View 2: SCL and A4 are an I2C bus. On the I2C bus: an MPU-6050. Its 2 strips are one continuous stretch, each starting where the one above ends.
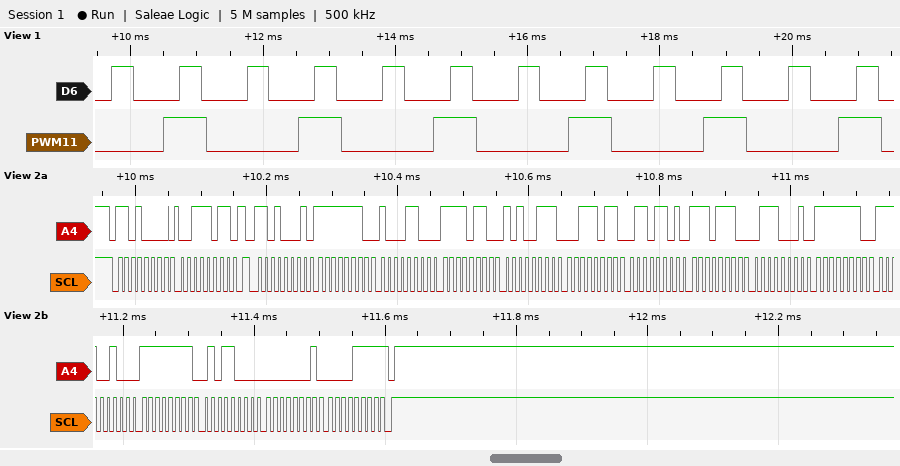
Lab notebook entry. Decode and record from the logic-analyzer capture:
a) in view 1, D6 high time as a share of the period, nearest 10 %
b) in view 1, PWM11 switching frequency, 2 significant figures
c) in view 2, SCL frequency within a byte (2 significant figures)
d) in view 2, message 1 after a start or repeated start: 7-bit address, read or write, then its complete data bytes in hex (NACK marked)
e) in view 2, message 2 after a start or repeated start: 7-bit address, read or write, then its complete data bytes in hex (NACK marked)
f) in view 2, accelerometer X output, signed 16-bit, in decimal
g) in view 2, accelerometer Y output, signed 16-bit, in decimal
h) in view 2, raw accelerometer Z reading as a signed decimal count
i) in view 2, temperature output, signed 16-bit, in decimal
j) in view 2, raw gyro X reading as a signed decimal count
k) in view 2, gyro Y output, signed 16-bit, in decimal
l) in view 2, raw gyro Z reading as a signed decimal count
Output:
30 %
490 Hz
100 kHz
0x68 write: 3B
0x68 read: FE 8C F6 A7 3B 6D EE 71 FE E4 FF 58 01 0F NACK
-372
-2393
15213
-4495
-284
-168
271
